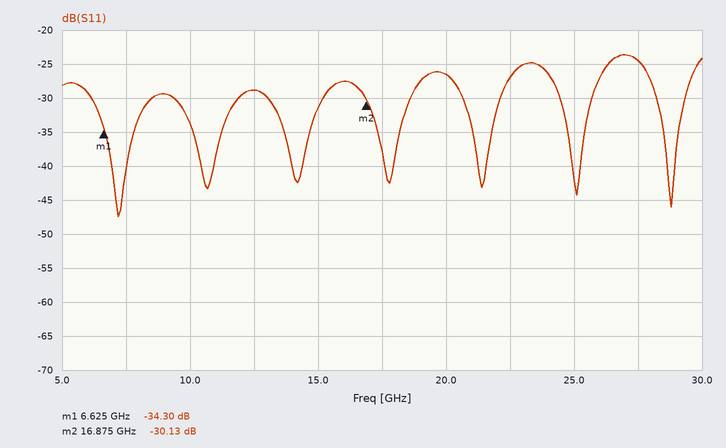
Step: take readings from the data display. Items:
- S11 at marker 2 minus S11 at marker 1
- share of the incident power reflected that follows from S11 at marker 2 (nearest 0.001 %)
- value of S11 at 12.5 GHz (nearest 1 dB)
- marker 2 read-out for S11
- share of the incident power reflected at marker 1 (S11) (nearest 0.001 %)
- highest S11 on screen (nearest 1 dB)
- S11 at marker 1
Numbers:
4.17 dB
0.097 %
-29 dB
-30.13 dB
0.037 %
-24 dB
-34.30 dB
